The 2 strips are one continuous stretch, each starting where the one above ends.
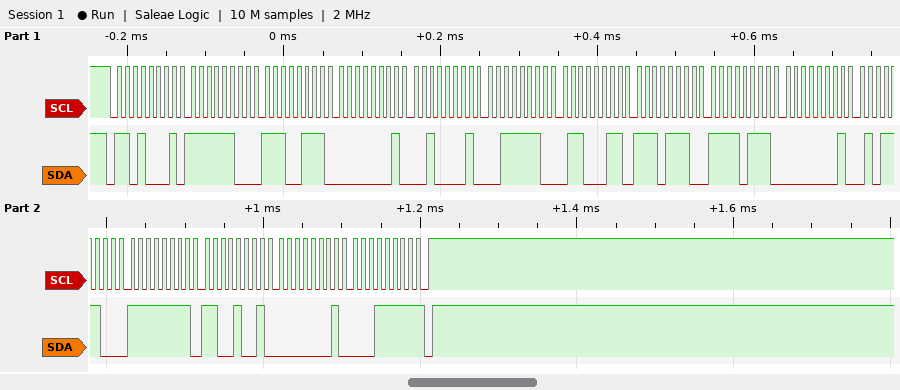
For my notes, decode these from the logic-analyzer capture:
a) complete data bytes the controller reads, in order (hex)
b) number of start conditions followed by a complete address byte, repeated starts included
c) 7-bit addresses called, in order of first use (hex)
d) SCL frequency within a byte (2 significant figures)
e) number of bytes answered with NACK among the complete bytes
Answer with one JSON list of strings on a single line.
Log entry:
["FC E7 01 21 3E 63 EE F7 01 5C FF C9 01 1F", "1", "0x68", "100 kHz", "1"]
